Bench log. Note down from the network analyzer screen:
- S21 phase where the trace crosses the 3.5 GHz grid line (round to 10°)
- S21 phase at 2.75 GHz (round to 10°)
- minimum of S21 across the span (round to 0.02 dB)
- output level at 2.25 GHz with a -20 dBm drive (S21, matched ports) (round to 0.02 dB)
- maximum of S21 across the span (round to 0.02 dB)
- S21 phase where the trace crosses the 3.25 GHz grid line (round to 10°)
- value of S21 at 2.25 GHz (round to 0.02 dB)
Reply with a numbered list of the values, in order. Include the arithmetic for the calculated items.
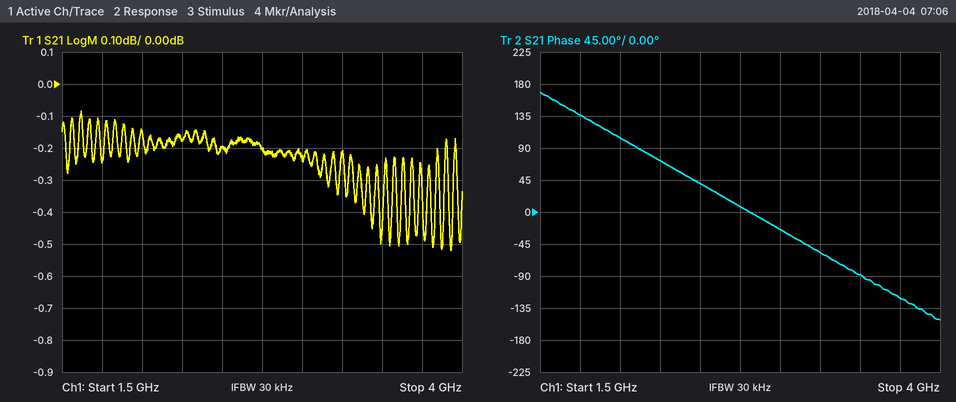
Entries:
1. -90°
2. 10°
3. -0.52 dB
4. -20 dBm + (-0.18 dB) = -20.18 dBm
5. -0.08 dB
6. -60°
7. -0.18 dB
